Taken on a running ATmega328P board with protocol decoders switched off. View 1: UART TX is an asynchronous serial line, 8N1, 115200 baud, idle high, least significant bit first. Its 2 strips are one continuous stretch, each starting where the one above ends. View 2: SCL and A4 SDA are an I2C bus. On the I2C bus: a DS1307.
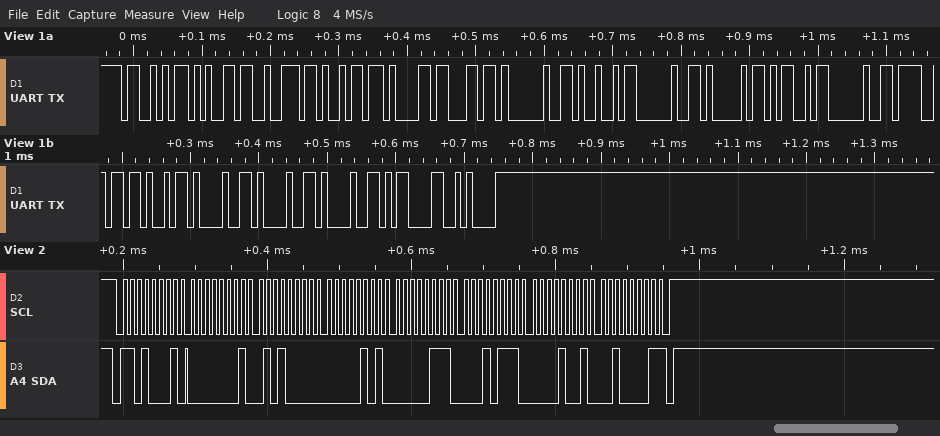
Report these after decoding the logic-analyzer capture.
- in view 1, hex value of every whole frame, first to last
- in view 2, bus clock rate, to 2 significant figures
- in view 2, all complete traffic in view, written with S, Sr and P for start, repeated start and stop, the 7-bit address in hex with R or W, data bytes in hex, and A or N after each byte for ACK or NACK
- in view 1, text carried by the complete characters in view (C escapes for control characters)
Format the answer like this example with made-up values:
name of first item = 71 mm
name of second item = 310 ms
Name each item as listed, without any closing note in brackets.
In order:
in view 1, hex value of every whole frame, first to last = 53 65 72 69 61 6C 20 49 20 41 4D 20 4F 4B 21 21 21 0D 0A
in view 2, bus clock rate, to 2 significant figures = 100 kHz
in view 2, all complete traffic in view, written with S, Sr and P for start, repeated start and stop, the 7-bit address in hex with R or W, data bytes in hex, and A or N after each byte for ACK or NACK = S 68R A 01 A 50 A 05 A 07 A 17 A 09 A 21 N P
in view 1, text carried by the complete characters in view = "Serial I AM OK!!!\r\n"
